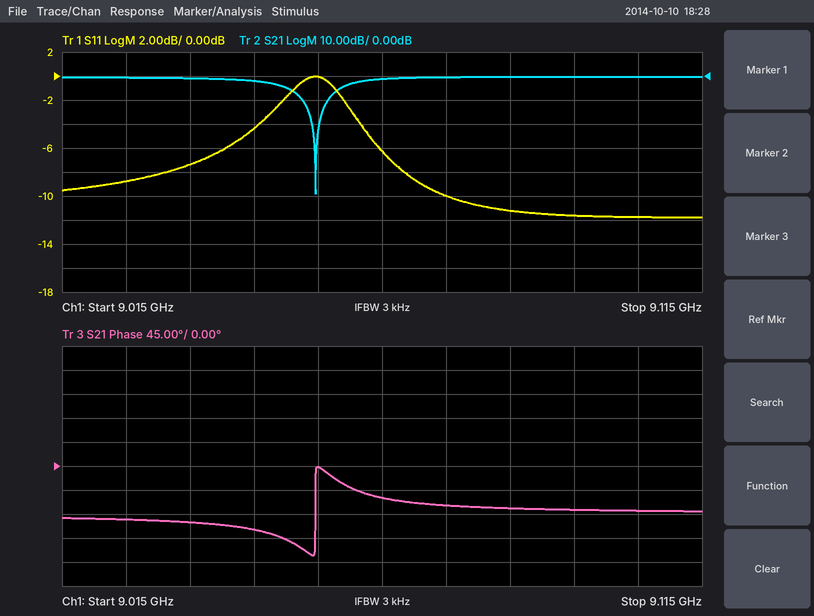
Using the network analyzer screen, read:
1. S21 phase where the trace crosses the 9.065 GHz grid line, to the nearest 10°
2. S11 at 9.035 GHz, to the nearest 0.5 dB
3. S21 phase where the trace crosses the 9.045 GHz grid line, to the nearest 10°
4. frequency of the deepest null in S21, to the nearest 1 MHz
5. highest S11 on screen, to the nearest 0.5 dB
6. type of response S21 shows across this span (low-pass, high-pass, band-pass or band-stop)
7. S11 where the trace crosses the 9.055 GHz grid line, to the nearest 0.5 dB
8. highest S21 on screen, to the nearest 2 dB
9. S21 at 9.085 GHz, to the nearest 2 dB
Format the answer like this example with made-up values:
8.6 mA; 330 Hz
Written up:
-60°; -7.5 dB; -120°; 9.055 GHz; 0.0 dB; band-stop; 0.0 dB; 0 dB; 0 dB
